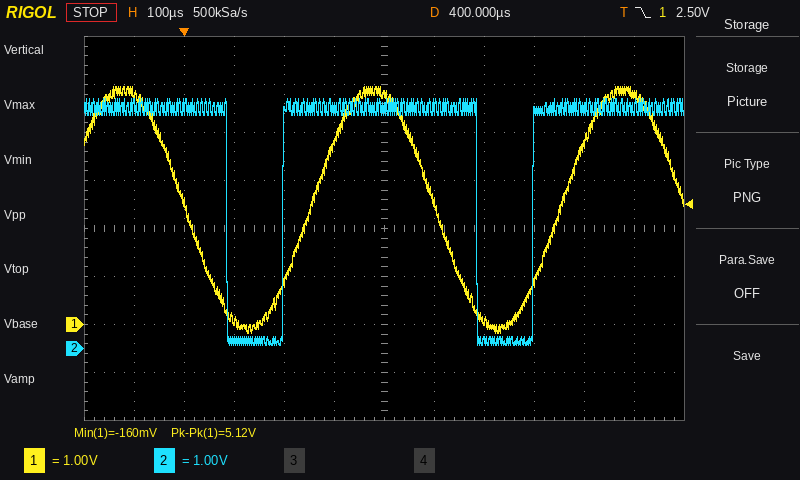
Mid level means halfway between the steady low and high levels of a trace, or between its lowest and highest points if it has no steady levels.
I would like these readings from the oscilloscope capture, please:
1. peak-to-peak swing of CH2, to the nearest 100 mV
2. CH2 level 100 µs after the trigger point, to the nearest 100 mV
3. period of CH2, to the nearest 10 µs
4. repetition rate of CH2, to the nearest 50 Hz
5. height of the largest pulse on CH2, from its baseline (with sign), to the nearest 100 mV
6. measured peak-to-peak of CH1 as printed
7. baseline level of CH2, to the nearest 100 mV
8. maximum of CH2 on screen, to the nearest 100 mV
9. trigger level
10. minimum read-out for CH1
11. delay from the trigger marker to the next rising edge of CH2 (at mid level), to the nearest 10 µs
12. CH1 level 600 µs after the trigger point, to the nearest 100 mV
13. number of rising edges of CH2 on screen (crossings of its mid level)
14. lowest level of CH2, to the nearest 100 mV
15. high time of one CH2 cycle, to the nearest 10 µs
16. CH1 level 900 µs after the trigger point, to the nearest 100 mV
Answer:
5.1 V
200 mV
500 µs
2.00 kHz
-4.9 V
5.12 V
5.0 V
5.2 V
2.50 V
-160 mV
200 µs
100 mV
2
100 mV
390 µs
4.8 V
